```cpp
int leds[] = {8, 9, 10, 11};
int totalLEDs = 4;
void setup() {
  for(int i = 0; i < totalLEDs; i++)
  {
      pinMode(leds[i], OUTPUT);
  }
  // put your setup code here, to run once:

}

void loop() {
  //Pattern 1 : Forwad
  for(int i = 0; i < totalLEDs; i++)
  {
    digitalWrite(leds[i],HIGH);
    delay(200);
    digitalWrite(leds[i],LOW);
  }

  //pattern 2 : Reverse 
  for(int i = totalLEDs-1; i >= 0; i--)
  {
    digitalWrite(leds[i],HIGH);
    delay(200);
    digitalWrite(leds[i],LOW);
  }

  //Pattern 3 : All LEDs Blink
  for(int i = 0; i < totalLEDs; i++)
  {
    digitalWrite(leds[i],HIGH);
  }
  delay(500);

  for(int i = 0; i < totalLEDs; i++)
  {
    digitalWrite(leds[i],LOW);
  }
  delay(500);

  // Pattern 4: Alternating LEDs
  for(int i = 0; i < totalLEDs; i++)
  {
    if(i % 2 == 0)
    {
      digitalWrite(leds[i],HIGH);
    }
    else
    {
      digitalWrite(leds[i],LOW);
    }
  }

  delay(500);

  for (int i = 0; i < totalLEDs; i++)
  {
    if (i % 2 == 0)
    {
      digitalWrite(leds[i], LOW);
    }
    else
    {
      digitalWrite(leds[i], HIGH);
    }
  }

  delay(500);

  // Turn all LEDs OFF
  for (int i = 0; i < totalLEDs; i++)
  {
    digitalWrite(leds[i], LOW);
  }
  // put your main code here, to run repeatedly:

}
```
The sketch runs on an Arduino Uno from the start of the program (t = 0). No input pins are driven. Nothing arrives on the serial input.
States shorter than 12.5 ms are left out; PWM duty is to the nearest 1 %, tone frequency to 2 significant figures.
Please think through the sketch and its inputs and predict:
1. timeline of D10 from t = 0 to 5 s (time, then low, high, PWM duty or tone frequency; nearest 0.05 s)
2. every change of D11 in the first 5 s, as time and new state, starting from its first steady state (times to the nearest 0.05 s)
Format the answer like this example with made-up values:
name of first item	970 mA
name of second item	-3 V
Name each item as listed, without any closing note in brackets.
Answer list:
timeline of D10 from t = 0 to 5 s	0 s low; 0.4 s high; 0.6 s low; 1 s high; 1.2 s low; 1.6 s high; 2.1 s low; 2.6 s high; 3.1 s low; 4 s high; 4.2 s low; 4.6 s high; 4.8 s low
every change of D11 in the first 5 s, as time and new state, starting from its first steady state	0 s low; 0.6 s high; 1 s low; 1.6 s high; 2.1 s low; 3.1 s high; 3.6 s low; 4.2 s high; 4.6 s low
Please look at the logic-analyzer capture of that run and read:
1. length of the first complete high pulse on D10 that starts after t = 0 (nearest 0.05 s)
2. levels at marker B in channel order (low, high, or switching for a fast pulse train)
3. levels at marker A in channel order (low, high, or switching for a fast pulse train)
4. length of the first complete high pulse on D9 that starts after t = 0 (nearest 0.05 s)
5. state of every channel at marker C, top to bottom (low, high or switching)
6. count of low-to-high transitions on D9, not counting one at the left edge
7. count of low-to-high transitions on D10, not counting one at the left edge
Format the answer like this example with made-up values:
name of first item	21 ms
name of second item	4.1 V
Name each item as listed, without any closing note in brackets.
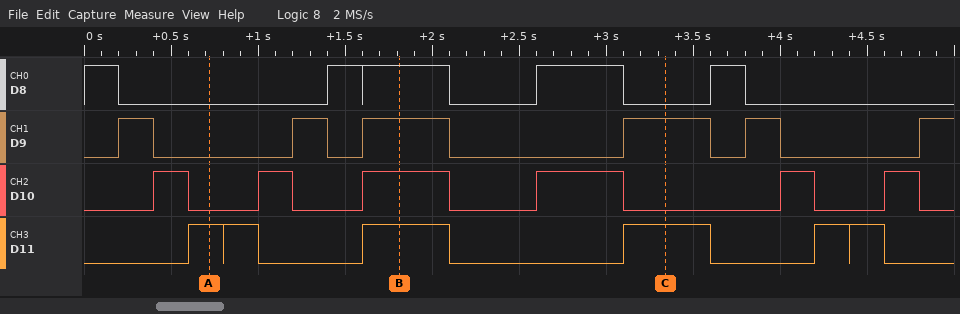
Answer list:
length of the first complete high pulse on D10 that starts after t = 0	0.20 s
levels at marker B in channel order	D8 high, D9 high, D10 high, D11 high
levels at marker A in channel order	D8 low, D9 low, D10 low, D11 high
length of the first complete high pulse on D9 that starts after t = 0	0.20 s
state of every channel at marker C, top to bottom	D8 low, D9 high, D10 low, D11 high
count of low-to-high transitions on D9, not counting one at the left edge	6
count of low-to-high transitions on D10, not counting one at the left edge	6
